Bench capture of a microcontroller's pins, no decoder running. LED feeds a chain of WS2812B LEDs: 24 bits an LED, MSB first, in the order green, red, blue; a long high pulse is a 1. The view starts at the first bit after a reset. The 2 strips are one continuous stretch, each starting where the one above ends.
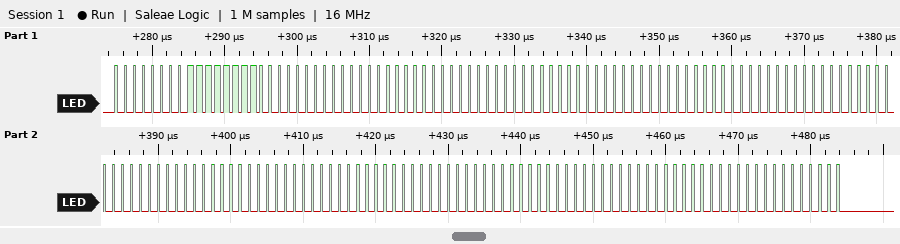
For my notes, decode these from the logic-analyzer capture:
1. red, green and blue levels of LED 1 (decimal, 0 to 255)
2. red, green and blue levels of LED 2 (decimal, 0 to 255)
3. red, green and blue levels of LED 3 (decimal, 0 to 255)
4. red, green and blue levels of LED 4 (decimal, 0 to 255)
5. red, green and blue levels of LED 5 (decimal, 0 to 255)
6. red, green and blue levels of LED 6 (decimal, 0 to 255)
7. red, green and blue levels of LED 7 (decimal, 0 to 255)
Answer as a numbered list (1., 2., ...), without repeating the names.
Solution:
1. 255, 0, 0
2. 0, 0, 0
3. 0, 0, 0
4. 0, 0, 0
5. 0, 0, 0
6. 0, 0, 0
7. 0, 0, 0
